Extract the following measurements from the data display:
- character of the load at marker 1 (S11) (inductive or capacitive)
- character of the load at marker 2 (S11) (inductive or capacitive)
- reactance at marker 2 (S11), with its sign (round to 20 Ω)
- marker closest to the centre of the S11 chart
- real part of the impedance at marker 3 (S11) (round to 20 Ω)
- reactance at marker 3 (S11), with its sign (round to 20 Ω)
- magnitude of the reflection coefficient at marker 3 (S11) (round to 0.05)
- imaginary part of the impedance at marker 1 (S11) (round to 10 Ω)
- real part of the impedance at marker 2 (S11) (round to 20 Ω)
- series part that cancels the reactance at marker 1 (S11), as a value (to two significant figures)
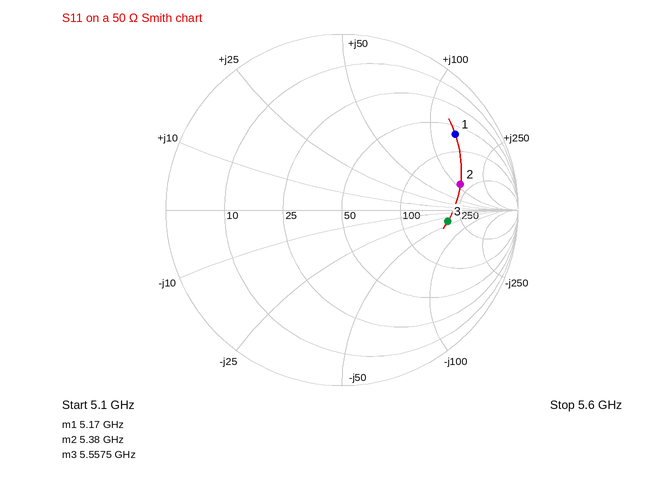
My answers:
inductive
inductive
+120 Ω
marker 3
200 Ω
-40 Ω
0.60
+140 Ω
200 Ω
220 fF
